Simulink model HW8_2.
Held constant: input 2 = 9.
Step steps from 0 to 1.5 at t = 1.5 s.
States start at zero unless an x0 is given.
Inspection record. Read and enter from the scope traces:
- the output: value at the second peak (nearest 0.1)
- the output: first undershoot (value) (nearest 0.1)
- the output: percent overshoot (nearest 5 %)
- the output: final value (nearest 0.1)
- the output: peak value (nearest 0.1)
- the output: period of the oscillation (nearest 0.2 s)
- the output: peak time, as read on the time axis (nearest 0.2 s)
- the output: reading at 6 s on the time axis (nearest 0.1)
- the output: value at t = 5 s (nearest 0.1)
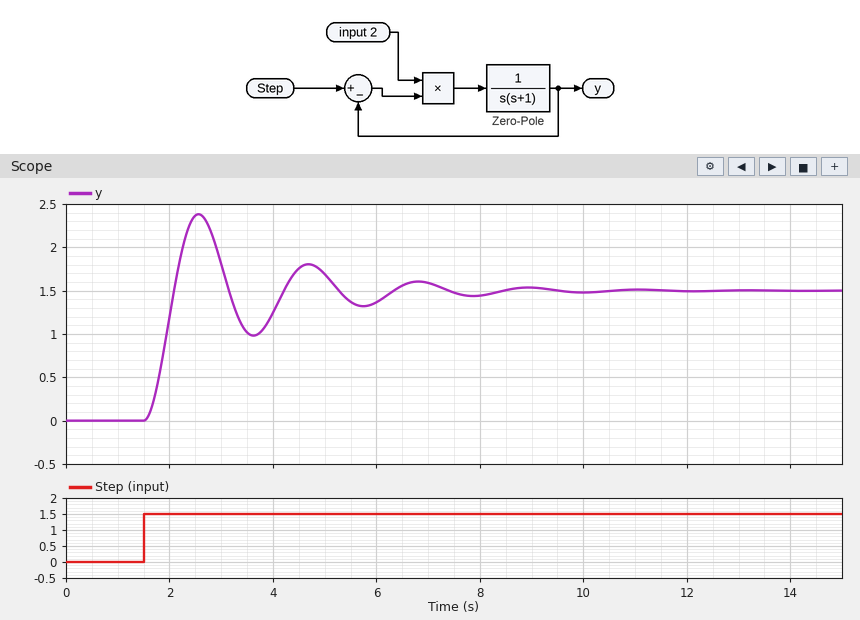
1.8
1.0
60 %
1.5
2.4
2.2 s
2.6 s
1.4
1.7
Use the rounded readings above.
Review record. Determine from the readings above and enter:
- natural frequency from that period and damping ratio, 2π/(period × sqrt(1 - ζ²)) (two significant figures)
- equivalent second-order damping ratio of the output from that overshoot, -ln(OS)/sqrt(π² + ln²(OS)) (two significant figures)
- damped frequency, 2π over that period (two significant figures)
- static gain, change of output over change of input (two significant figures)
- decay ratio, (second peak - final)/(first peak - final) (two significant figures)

2.9 rad/s
0.16
2.9 rad/s
1.0
0.33
